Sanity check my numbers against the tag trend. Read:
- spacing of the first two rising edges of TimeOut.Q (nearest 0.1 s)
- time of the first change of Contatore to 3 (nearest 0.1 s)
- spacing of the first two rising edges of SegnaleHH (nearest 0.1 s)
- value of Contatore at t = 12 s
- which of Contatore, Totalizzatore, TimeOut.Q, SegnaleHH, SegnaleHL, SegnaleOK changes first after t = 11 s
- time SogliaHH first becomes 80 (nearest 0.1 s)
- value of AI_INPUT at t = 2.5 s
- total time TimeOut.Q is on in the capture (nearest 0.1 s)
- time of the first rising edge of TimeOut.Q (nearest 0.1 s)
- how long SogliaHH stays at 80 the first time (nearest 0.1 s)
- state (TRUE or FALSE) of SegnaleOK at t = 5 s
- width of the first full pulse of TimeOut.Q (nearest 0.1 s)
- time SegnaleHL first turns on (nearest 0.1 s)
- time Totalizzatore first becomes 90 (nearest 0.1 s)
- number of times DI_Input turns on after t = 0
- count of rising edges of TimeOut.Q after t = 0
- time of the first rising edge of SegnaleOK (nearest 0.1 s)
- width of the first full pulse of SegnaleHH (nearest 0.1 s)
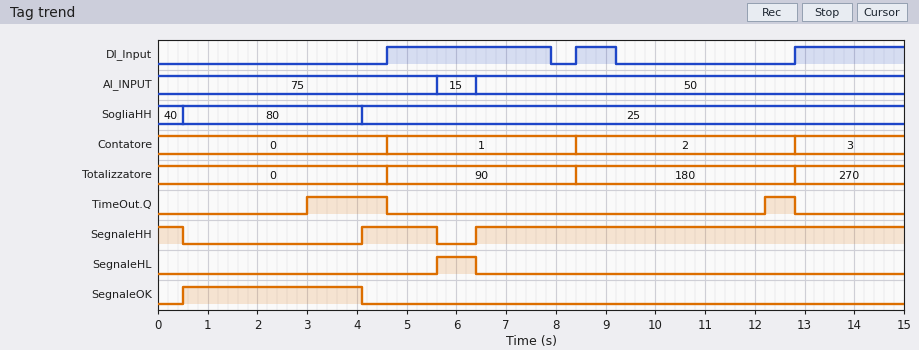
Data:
9.2 s
12.8 s
2.3 s
2
TimeOut.Q
0.5 s
75
2.2 s
3.0 s
3.6 s
FALSE
1.6 s
5.6 s
4.6 s
3
2
0.5 s
1.5 s
